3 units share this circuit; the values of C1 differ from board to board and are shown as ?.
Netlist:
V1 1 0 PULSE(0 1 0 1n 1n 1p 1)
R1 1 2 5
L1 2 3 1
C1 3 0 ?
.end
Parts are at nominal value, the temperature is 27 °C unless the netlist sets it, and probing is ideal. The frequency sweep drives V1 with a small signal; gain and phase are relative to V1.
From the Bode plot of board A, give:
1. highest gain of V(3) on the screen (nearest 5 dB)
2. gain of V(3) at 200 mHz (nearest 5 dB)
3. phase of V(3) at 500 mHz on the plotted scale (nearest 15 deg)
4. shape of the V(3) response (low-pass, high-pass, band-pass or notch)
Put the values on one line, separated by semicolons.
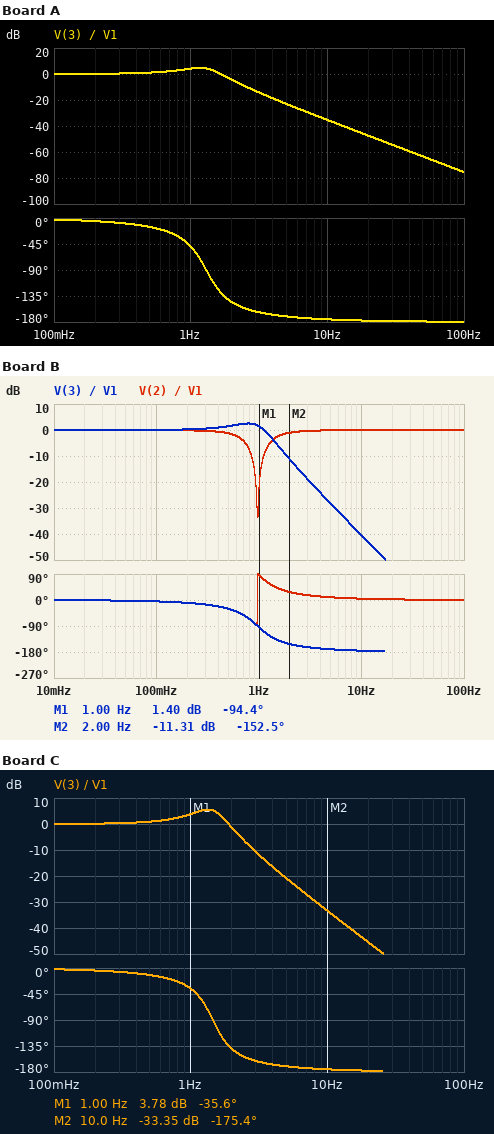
5 dB; 0 dB; -15 deg; low-pass
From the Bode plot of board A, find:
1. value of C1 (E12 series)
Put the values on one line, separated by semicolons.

15 mF
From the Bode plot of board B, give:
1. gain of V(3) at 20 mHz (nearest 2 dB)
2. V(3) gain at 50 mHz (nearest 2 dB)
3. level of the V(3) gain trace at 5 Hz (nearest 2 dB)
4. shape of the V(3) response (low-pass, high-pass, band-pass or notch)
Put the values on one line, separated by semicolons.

0 dB; 0 dB; -28 dB; low-pass
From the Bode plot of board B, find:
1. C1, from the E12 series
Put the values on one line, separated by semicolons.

27 mF
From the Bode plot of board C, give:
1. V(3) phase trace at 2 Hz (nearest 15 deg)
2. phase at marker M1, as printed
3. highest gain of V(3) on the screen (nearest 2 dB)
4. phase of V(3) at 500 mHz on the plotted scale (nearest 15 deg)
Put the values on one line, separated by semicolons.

-135 deg; -35.6 deg; 6 dB; -15 deg
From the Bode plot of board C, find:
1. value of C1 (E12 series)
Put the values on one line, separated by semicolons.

12 mF
